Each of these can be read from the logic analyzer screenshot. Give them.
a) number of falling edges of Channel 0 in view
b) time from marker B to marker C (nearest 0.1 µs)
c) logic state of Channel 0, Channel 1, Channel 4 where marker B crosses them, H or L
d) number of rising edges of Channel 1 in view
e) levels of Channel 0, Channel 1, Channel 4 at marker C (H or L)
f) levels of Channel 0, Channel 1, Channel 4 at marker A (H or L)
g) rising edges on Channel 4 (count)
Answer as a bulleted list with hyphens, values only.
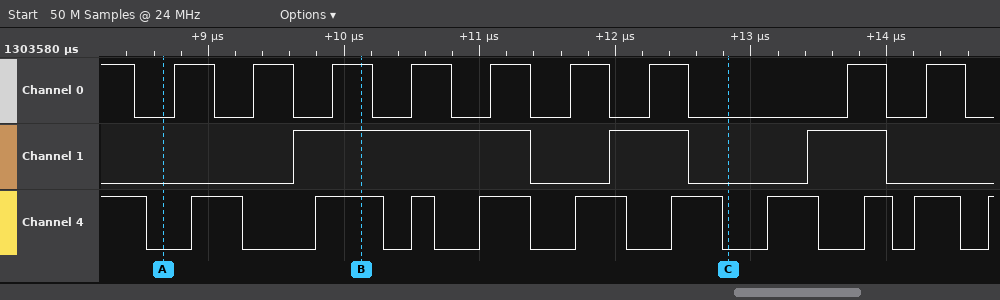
- 10
- 2.7 µs
- Channel 0=H, Channel 1=H, Channel 4=H
- 3
- Channel 0=L, Channel 1=L, Channel 4=L
- Channel 0=L, Channel 1=L, Channel 4=L
- 10
